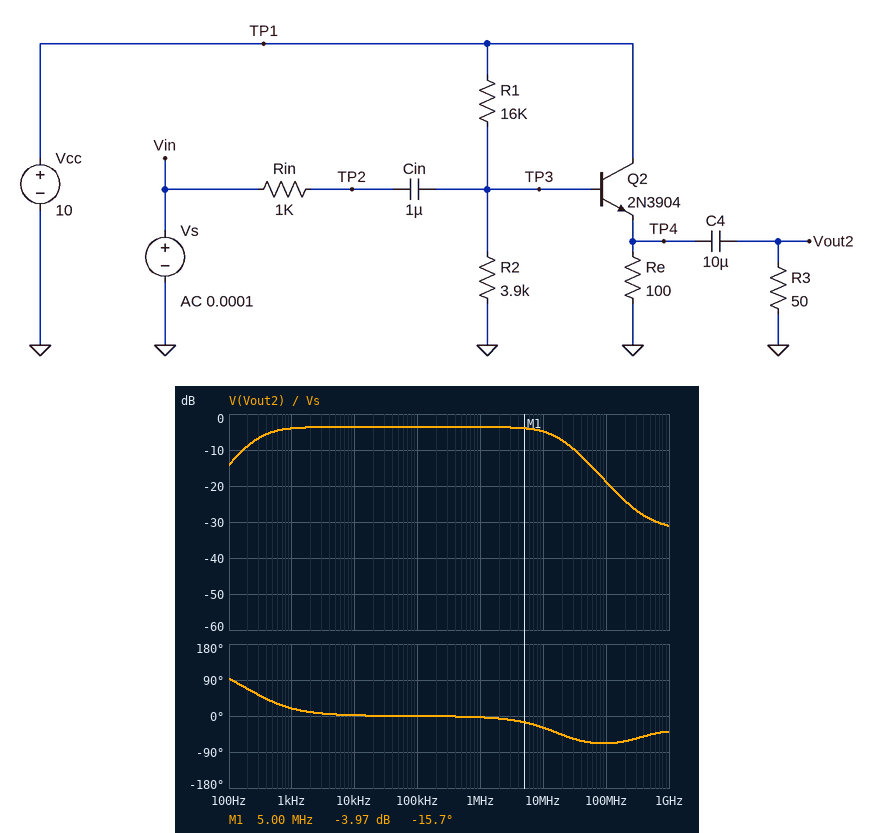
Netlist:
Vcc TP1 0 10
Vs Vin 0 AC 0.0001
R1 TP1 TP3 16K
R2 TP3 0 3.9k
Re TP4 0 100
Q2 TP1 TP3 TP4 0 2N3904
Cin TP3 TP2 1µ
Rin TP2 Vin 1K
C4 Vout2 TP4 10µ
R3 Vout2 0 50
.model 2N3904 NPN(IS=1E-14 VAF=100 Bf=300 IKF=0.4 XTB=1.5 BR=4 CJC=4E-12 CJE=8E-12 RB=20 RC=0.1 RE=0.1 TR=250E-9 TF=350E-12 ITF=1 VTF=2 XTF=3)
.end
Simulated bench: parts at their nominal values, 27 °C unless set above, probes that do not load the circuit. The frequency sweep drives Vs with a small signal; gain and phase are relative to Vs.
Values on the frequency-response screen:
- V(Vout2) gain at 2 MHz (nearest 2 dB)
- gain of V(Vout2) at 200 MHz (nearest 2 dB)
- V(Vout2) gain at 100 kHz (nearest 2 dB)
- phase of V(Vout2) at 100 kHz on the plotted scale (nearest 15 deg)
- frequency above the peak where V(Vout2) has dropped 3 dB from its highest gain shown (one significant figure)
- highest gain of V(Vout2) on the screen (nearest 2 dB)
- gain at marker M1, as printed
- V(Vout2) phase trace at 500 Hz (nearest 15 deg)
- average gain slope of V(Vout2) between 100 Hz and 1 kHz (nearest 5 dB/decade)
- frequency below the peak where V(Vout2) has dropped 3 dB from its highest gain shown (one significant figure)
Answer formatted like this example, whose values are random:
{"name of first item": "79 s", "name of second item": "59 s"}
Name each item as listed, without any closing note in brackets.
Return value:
{"V(Vout2) gain at 2 MHz": "-4 dB", "gain of V(Vout2) at 200 MHz": "-24 dB", "V(Vout2) gain at 100 kHz": "-4 dB", "phase of V(Vout2) at 100 kHz on the plotted scale": "0 deg", "frequency above the peak where V(Vout2) has dropped 3 dB from its highest gain shown": "20 MHz", "highest gain of V(Vout2) on the screen": "-4 dB", "gain at marker M1, as printed": "-3.97 dB", "V(Vout2) phase trace at 500 Hz": "30 deg", "average gain slope of V(Vout2) between 100 Hz and 1 kHz": "10 dB/decade", "frequency below the peak where V(Vout2) has dropped 3 dB from its highest gain shown": "300 Hz"}
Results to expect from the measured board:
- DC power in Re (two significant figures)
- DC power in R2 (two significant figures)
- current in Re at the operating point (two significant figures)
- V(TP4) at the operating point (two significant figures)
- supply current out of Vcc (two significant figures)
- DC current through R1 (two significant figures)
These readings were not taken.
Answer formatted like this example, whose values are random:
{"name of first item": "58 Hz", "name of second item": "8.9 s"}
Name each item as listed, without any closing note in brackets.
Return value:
{"DC power in Re": "13 mW", "DC power in R2": "880 µW", "current in Re at the operating point": "11 mA", "V(TP4) at the operating point": "1.1 V", "supply current out of Vcc": "12 mA", "DC current through R1": "510 µA"}
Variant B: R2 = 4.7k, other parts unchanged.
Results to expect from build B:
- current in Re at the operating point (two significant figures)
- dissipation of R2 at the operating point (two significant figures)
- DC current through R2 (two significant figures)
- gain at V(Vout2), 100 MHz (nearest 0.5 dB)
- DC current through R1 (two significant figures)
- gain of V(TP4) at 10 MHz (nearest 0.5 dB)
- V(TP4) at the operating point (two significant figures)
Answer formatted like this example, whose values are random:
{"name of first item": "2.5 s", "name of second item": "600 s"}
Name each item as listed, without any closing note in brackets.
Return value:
{"current in Re at the operating point": "14 mA", "dissipation of R2 at the operating point": "950 µW", "DC current through R2": "450 µA", "gain at V(Vout2), 100 MHz": "-18.5 dB", "DC current through R1": "490 µA", "gain of V(TP4) at 10 MHz": "-4.5 dB", "V(TP4) at the operating point": "1.4 V"}
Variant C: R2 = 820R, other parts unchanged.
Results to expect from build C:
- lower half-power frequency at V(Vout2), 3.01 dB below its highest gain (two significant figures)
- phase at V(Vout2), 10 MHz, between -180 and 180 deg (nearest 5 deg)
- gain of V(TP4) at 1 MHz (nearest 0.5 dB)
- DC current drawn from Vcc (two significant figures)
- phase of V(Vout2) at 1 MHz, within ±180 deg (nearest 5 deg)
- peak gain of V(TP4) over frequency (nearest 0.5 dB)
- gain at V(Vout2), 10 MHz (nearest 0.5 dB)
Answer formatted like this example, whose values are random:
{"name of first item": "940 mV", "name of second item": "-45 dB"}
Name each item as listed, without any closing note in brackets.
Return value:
{"lower half-power frequency at V(Vout2), 3.01 dB below its highest gain": "25 MHz", "phase at V(Vout2), 10 MHz, between -180 and 180 deg": "65 deg", "gain of V(TP4) at 1 MHz": "-57.0 dB", "DC current drawn from Vcc": "600 µA", "phase of V(Vout2) at 1 MHz, within ±180 deg": "45 deg", "peak gain of V(TP4) over frequency": "-31.5 dB", "gain at V(Vout2), 10 MHz": "-40.5 dB"}
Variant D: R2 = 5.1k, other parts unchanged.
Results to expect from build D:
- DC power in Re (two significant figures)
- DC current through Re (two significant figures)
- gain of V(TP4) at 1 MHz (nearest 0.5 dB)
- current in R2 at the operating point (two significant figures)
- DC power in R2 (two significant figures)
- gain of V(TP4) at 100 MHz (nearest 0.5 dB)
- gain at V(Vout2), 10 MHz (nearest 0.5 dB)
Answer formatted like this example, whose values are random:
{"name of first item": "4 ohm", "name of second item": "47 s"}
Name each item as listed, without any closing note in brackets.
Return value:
{"DC power in Re": "23 mW", "DC current through Re": "15 mA", "gain of V(TP4) at 1 MHz": "-3.0 dB", "current in R2 at the operating point": "440 µA", "DC power in R2": "980 µW", "gain of V(TP4) at 100 MHz": "-18.5 dB", "gain at V(Vout2), 10 MHz": "-4.5 dB"}
